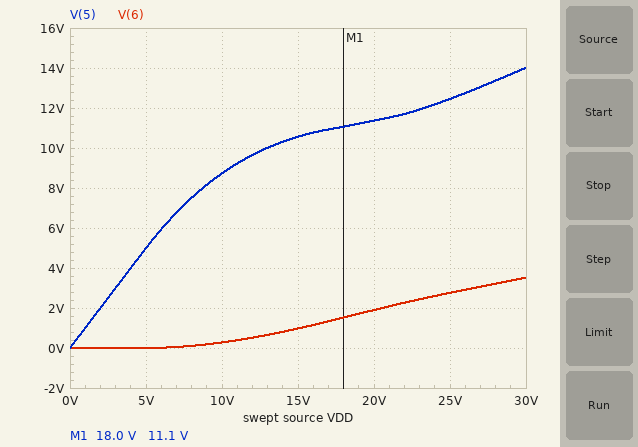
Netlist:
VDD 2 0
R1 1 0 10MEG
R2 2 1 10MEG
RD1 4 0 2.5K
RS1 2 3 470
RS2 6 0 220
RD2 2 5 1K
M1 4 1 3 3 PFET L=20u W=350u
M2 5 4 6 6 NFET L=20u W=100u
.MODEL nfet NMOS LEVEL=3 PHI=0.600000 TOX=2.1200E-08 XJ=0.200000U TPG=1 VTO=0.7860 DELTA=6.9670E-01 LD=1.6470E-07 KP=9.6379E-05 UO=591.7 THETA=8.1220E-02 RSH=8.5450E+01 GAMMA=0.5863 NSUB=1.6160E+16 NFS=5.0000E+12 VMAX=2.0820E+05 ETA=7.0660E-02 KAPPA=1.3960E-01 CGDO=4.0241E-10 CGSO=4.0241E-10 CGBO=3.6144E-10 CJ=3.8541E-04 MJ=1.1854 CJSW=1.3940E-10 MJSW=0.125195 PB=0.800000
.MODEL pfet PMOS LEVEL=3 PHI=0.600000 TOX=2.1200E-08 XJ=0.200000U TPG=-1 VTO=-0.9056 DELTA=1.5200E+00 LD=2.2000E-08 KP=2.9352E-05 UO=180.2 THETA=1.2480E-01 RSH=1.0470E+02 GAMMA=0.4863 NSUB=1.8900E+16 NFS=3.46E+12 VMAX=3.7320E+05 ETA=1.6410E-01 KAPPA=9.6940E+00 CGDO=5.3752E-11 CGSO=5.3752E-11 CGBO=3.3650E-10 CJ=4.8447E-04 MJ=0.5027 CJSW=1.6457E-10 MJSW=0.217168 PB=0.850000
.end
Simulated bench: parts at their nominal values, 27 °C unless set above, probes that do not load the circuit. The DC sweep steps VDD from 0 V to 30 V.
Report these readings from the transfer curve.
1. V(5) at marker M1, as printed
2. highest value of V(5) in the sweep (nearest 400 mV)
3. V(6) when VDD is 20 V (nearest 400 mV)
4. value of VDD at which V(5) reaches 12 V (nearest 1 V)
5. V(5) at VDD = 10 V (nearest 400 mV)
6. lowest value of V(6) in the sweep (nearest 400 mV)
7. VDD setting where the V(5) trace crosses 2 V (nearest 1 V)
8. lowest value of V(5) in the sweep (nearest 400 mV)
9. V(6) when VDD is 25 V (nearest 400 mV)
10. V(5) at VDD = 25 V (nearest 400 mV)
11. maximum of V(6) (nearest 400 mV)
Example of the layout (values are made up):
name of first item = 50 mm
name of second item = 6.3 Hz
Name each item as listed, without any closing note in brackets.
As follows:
V(5) at marker M1, as printed = 11.1 V
highest value of V(5) in the sweep = 14.0 V
V(6) when VDD is 20 V = 2.0 V
value of VDD at which V(5) reaches 12 V = 23 V
V(5) at VDD = 10 V = 8.8 V
lowest value of V(6) in the sweep = 0 V
VDD setting where the V(5) trace crosses 2 V = 2 V
lowest value of V(5) in the sweep = 0 V
V(6) when VDD is 25 V = 2.8 V
V(5) at VDD = 25 V = 12.4 V
maximum of V(6) = 3.6 V
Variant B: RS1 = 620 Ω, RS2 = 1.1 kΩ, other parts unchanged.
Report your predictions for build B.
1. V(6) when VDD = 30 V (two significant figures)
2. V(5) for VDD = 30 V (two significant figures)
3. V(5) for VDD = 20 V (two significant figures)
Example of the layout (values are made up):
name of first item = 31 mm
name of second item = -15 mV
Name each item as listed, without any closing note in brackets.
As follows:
V(6) when VDD = 30 V = 8.8 V
V(5) for VDD = 30 V = 22 V
V(5) for VDD = 20 V = 16 V
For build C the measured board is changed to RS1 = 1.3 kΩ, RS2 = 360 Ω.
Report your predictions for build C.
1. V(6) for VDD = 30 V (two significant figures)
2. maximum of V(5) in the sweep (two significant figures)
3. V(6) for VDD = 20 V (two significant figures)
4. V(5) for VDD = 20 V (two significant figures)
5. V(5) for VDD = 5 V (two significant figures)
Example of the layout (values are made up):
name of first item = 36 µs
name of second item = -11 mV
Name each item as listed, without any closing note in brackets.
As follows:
V(6) for VDD = 30 V = 3.1 V
maximum of V(5) in the sweep = 21 V
V(6) for VDD = 20 V = 1.4 V
V(5) for VDD = 20 V = 16 V
V(5) for VDD = 5 V = 5.0 V
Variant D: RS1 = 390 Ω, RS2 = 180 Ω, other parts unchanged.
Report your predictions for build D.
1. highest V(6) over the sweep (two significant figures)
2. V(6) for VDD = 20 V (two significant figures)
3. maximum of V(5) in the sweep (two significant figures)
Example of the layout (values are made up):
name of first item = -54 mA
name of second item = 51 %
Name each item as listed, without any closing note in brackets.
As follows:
highest V(6) over the sweep = 3.0 V
V(6) for VDD = 20 V = 1.7 V
maximum of V(5) in the sweep = 13 V
